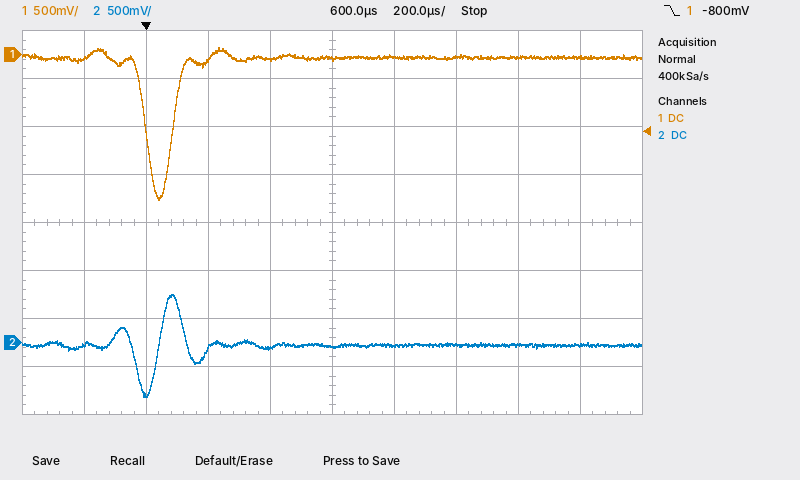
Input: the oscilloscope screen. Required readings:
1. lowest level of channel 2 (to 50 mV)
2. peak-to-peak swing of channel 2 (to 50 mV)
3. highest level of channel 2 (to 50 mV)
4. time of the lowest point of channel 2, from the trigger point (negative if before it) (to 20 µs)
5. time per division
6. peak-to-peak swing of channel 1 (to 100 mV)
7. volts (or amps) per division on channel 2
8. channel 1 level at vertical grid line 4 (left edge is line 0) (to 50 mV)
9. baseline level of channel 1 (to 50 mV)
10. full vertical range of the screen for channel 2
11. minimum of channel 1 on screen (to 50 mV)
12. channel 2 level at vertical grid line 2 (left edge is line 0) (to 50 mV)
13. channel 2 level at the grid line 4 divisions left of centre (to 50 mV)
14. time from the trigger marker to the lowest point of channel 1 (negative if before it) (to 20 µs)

-550 mV
1.05 V
500 mV
0 µs
200 µs
1.60 V
500 mV
-50 mV
-50 mV
4 V
-1.50 V
-550 mV
0 mV
+40 µs
